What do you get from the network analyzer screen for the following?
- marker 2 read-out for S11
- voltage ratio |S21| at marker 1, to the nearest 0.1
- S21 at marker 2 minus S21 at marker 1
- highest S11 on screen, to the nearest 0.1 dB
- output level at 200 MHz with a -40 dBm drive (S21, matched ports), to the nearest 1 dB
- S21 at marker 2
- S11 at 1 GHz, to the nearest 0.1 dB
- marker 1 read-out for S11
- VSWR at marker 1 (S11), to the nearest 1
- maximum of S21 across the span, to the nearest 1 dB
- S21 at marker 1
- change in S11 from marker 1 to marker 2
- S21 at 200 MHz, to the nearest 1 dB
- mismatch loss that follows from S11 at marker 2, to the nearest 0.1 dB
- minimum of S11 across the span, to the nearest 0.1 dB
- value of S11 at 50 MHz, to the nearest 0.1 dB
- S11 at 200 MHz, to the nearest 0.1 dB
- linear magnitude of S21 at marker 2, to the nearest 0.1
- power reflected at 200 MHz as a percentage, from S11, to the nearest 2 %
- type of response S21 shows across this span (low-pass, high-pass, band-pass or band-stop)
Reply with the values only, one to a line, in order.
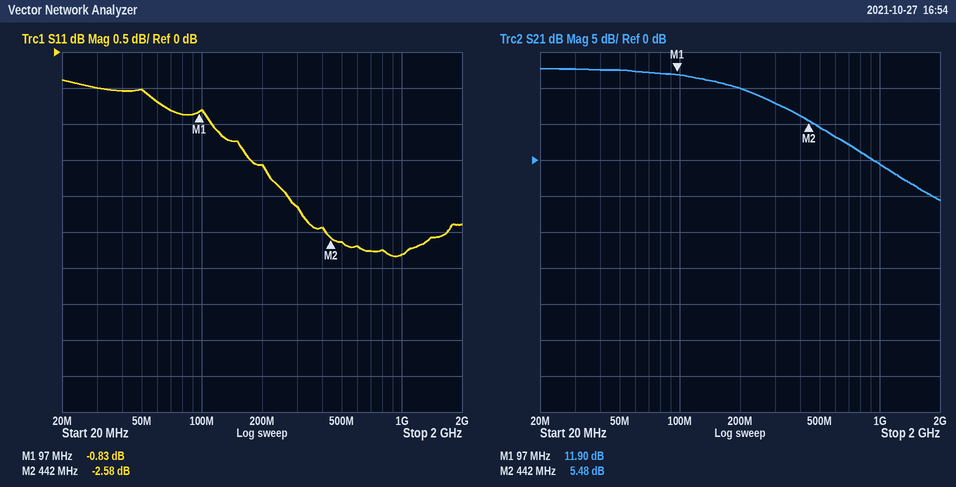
-2.58 dB
3.9
-6.42 dB
-0.4 dB
-30 dBm
5.48 dB
-2.8 dB
-0.83 dB
21
13 dB
11.90 dB
-1.75 dB
10 dB
3.5 dB
-2.8 dB
-0.5 dB
-1.6 dB
1.9
70 %
low-pass
